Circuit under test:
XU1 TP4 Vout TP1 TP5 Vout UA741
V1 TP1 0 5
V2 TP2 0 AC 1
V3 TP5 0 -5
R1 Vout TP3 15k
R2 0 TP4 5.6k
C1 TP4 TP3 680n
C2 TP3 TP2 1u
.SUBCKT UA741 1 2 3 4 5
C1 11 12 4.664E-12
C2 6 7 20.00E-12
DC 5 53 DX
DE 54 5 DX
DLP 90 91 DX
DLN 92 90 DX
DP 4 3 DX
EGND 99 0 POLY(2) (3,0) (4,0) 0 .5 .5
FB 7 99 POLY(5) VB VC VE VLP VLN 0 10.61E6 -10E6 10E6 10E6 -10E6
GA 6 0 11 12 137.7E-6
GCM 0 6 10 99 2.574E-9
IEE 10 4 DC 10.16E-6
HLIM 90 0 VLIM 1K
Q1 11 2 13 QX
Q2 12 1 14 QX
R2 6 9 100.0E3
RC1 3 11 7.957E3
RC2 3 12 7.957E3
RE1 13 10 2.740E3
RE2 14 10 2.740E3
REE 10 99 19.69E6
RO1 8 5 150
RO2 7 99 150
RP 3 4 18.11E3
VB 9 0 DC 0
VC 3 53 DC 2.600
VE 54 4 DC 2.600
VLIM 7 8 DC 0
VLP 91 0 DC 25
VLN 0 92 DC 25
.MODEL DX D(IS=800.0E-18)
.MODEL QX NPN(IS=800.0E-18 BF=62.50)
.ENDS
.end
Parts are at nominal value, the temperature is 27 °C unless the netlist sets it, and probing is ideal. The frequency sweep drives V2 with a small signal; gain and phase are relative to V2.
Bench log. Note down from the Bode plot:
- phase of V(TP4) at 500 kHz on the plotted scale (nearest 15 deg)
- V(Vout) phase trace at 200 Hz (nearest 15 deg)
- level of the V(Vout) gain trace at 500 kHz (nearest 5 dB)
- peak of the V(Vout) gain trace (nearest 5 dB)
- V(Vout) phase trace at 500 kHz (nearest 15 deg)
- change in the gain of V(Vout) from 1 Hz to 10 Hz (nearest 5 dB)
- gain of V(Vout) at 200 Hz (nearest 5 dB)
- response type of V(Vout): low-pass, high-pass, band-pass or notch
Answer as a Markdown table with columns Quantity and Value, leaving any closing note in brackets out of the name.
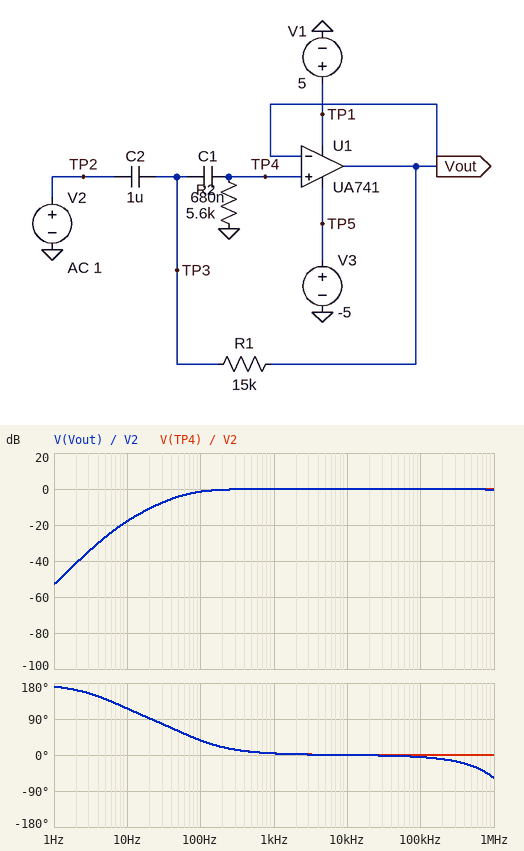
| Quantity | Value |
|---|---|
| phase of V(TP4) at 500 kHz on the plotted scale | 0 deg |
| V(Vout) phase trace at 200 Hz | 15 deg |
| level of the V(Vout) gain trace at 500 kHz | 0 dB |
| peak of the V(Vout) gain trace | 0 dB |
| V(Vout) phase trace at 500 kHz | -30 deg |
| change in the gain of V(Vout) from 1 Hz to 10 Hz | 35 dB |
| gain of V(Vout) at 200 Hz | 0 dB |
| response type of V(Vout): low-pass, high-pass, band-pass or notch | high-pass |
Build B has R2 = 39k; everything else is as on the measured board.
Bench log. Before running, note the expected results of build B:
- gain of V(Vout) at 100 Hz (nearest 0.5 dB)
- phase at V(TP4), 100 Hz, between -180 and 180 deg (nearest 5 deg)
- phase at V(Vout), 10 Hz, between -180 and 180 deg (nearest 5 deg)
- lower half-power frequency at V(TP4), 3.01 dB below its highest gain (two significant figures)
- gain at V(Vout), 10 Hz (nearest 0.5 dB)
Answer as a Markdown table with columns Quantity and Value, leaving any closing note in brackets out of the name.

| Quantity | Value |
|---|---|
| gain of V(Vout) at 100 Hz | 0 dB |
| phase at V(TP4), 100 Hz, between -180 and 180 deg | 5 deg |
| phase at V(Vout), 10 Hz, between -180 and 180 deg | 70 deg |
| lower half-power frequency at V(TP4), 3.01 dB below its highest gain | 7.3 Hz |
| gain at V(Vout), 10 Hz | -0.5 dB |
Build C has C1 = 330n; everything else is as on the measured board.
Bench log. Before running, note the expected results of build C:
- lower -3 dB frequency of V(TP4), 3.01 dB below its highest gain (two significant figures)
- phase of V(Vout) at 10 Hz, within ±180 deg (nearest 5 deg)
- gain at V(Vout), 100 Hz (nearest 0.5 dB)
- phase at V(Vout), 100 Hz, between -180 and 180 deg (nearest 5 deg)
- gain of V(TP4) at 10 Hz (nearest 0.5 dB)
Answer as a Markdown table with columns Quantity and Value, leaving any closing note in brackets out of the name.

| Quantity | Value |
|---|---|
| lower -3 dB frequency of V(TP4), 3.01 dB below its highest gain | 110 Hz |
| phase of V(Vout) at 10 Hz, within ±180 deg | 125 deg |
| gain at V(Vout), 100 Hz | -3.5 dB |
| phase at V(Vout), 100 Hz, between -180 and 180 deg | 50 deg |
| gain of V(TP4) at 10 Hz | -23.0 dB |
